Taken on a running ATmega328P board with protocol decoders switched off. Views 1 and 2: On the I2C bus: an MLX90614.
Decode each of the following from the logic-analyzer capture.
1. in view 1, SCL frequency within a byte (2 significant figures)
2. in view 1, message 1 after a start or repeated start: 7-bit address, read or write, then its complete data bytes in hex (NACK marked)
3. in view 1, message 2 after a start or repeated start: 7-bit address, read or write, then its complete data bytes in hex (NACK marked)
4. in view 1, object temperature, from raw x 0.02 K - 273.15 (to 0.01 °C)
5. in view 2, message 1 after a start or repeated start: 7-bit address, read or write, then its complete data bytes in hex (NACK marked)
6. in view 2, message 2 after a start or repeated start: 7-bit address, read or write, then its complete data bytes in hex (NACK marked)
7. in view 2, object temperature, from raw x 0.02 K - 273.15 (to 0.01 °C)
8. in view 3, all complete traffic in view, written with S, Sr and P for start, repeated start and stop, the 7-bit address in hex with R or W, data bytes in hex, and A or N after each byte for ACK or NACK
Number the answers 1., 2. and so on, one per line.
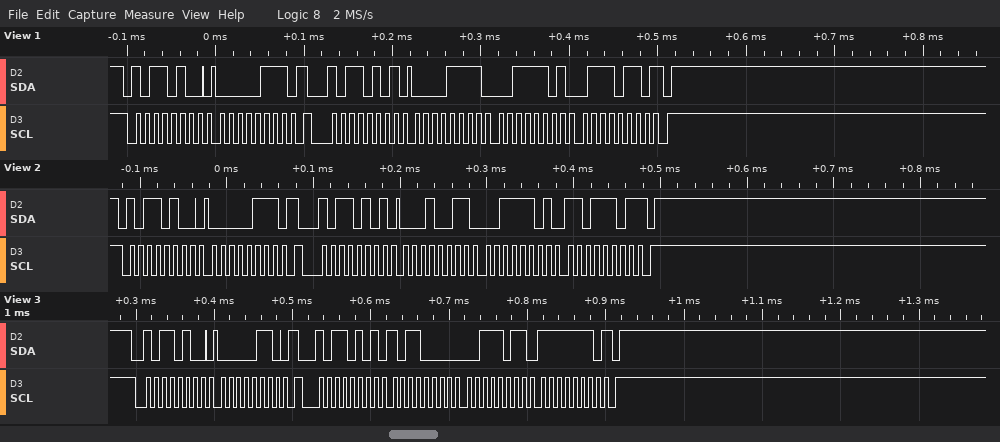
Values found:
1. 100 kHz
2. 0x5A write: 07
3. 0x5A read: 0F 3D 76 NACK
4. 39.47 °C
5. 0x5A write: 07
6. 0x5A read: 13 3D DD NACK
7. 39.55 °C
8. S 5AW A 06 A Sr 5AR A B0 A 3B A FE N P
